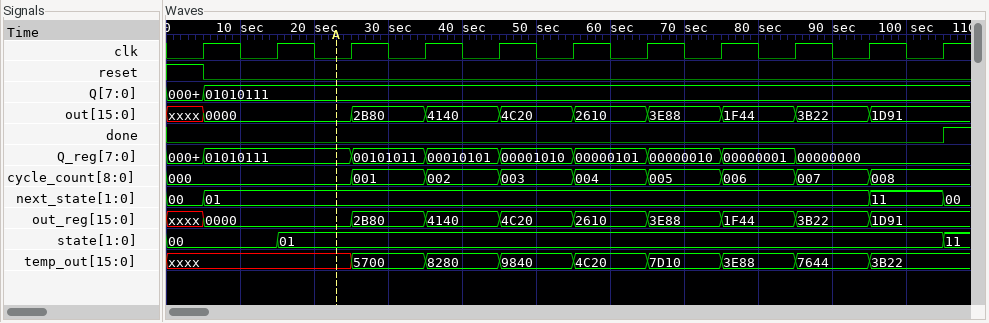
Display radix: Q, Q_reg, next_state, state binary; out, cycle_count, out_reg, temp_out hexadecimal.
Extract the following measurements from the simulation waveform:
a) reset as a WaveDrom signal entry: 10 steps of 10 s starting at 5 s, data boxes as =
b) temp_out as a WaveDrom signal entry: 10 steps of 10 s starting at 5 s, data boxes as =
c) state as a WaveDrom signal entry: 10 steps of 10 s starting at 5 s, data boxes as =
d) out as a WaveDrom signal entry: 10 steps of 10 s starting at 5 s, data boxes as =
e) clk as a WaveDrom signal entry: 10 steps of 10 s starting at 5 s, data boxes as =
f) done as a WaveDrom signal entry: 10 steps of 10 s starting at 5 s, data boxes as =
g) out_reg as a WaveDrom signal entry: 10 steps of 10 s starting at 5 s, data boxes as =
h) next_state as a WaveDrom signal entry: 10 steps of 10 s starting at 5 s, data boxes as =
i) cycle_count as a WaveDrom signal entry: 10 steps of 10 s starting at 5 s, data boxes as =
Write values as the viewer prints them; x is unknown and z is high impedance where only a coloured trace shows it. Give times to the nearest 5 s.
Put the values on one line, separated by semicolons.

{name: 'reset', wave: '0.........'}; {name: 'temp_out', wave: 'x.========', data: '5700 8280 9840 4C20 7D10 3E88 7644 3B22'}; {name: 'state', wave: '==........', data: '00 01'}; {name: 'out', wave: '=.========', data: '0000 2B80 4140 4C20 2610 3E88 1F44 3B22 1D91'}; {name: 'clk', wave: 'p.........'}; {name: 'done', wave: '0.........'}; {name: 'out_reg', wave: '=.========', data: '0000 2B80 4140 4C20 2610 3E88 1F44 3B22 1D91'}; {name: 'next_state', wave: '=........=', data: '01 11'}; {name: 'cycle_count', wave: '=.========', data: '000 001 002 003 004 005 006 007 008'}
